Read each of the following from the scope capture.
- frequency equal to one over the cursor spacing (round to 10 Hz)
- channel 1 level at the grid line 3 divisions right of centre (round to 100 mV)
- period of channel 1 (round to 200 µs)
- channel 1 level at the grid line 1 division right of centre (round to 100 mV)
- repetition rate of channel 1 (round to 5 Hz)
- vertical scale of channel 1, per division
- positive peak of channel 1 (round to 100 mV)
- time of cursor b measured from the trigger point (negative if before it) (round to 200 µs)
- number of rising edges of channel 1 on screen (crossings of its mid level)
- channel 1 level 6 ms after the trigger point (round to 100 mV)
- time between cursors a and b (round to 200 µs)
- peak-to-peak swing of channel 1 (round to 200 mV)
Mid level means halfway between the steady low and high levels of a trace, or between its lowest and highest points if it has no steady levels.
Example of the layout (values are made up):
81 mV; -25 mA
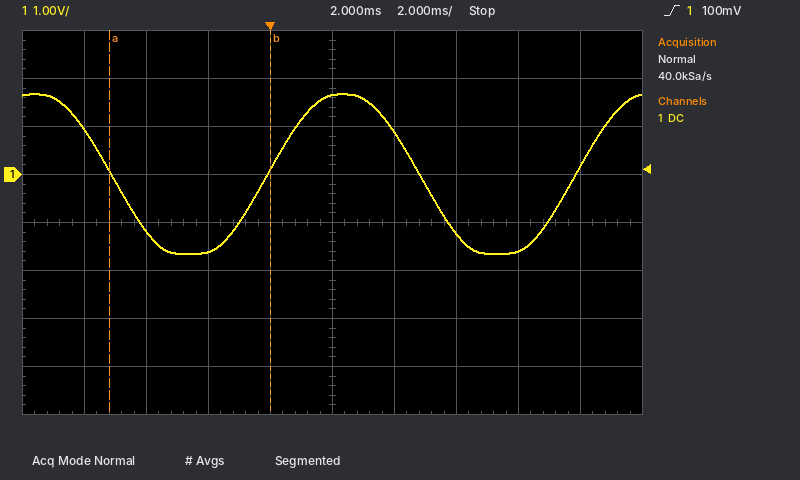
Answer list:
190 Hz; -1.6 V; 10.0 ms; 900 mV; 100 Hz; 1 V; 1.7 V; 0.0 ms; 2; -1.2 V; 5.2 ms; 3.4 V
